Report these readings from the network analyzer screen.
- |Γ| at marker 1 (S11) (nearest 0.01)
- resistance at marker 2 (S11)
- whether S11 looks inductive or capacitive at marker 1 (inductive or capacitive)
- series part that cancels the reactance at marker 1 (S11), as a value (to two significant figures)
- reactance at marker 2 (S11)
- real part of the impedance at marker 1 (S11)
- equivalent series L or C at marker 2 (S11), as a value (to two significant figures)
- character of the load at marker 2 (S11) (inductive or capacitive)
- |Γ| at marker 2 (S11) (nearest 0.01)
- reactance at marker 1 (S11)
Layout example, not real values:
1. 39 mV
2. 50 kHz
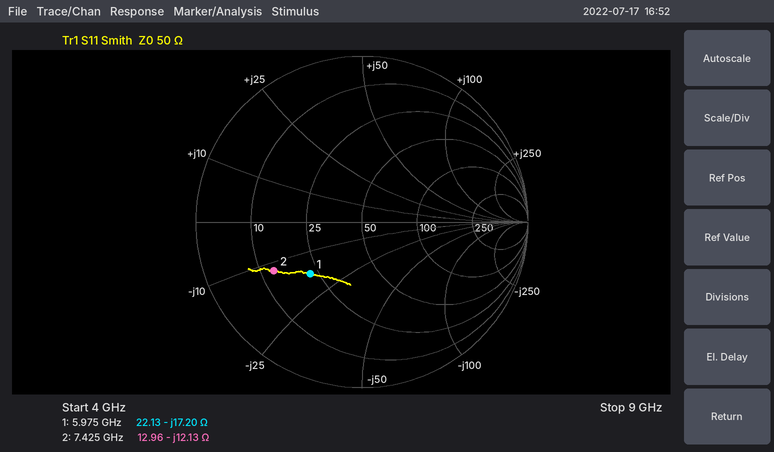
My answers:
1. 0.44
2. 12.96 Ω
3. capacitive
4. 460 pH
5. -12.13 Ω
6. 22.13 Ω
7. 1.8 pF
8. capacitive
9. 0.61
10. -17.20 Ω
